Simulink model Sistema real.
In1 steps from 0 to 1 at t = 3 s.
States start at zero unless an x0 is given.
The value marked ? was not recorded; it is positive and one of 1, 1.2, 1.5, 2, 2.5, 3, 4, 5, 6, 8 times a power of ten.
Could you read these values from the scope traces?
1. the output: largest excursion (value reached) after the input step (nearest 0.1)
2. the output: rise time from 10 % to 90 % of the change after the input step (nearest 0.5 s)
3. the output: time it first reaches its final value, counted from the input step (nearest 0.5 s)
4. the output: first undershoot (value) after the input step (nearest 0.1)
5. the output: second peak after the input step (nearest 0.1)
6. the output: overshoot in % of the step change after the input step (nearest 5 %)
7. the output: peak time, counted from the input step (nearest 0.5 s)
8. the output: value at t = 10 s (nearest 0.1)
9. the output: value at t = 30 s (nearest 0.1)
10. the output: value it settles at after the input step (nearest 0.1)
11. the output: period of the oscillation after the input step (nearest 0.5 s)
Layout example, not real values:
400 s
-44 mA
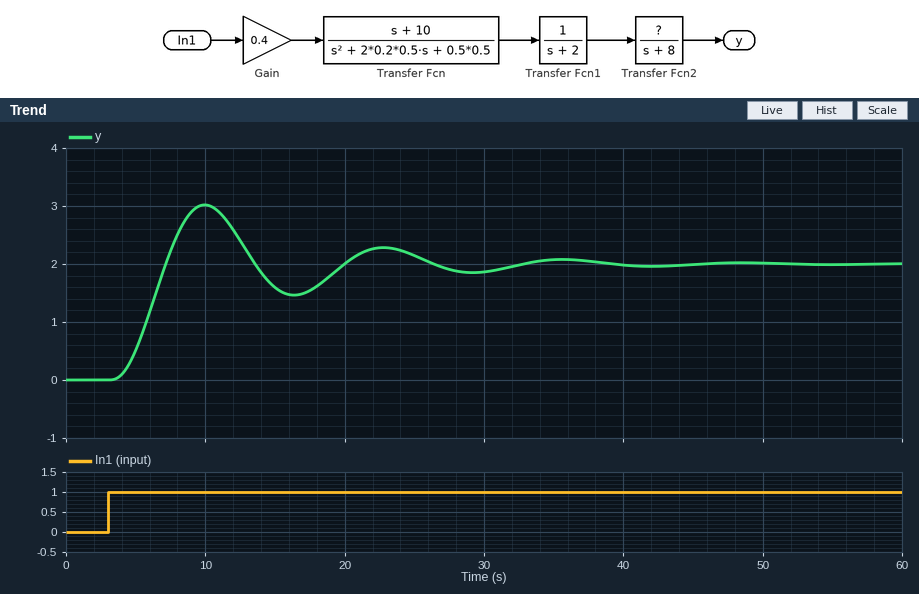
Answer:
3.0
2.5 s
4.0 s
1.5
2.3
50 %
7.0 s
3.0
1.9
2.0
13.0 s
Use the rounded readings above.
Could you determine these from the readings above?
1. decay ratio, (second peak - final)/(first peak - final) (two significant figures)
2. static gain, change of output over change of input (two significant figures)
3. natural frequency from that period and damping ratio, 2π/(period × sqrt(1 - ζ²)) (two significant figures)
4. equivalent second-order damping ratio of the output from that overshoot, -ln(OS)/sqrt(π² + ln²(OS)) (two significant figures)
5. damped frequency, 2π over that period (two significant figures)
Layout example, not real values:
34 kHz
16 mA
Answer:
0.30
2.0
0.50 rad/s
0.22
0.48 rad/s
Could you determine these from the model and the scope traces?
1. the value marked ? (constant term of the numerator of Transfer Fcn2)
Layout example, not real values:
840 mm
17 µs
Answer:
2
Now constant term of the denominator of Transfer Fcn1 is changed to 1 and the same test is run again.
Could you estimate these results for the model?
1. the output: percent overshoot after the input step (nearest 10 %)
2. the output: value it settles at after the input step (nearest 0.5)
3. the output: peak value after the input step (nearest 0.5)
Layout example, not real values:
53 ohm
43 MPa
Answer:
50 %
4.0
6.0
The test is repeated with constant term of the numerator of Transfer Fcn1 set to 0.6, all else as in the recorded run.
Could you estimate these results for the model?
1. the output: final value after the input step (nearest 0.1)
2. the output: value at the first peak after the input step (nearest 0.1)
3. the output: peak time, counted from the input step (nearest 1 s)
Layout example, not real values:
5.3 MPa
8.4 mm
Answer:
1.2
1.8
7 s
